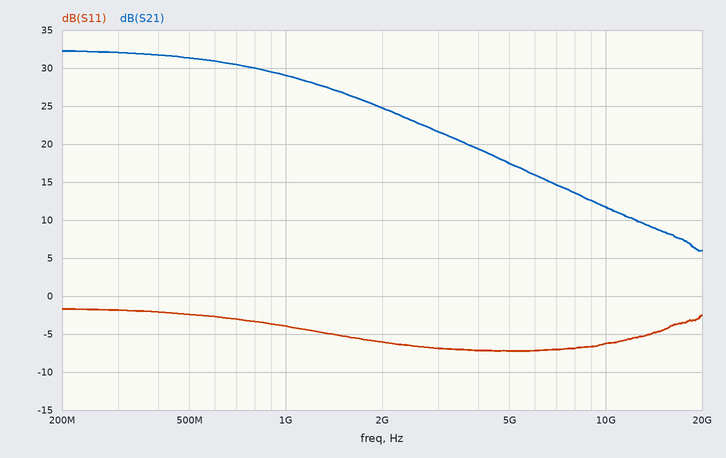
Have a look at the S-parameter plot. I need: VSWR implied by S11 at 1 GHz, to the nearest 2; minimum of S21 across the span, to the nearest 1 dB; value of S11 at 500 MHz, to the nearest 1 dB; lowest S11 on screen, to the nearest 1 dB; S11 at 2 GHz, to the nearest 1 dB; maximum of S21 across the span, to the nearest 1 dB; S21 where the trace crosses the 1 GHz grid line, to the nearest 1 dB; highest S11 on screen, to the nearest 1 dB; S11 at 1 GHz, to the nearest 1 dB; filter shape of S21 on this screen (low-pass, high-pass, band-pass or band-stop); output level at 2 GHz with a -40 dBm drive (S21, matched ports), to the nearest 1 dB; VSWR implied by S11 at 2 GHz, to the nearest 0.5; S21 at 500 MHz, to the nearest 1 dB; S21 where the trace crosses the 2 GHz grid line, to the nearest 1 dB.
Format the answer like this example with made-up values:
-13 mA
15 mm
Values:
4
6 dB
-2 dB
-7 dB
-6 dB
32 dB
29 dB
-2 dB
-4 dB
low-pass
-15 dBm
3.0
31 dB
25 dB
